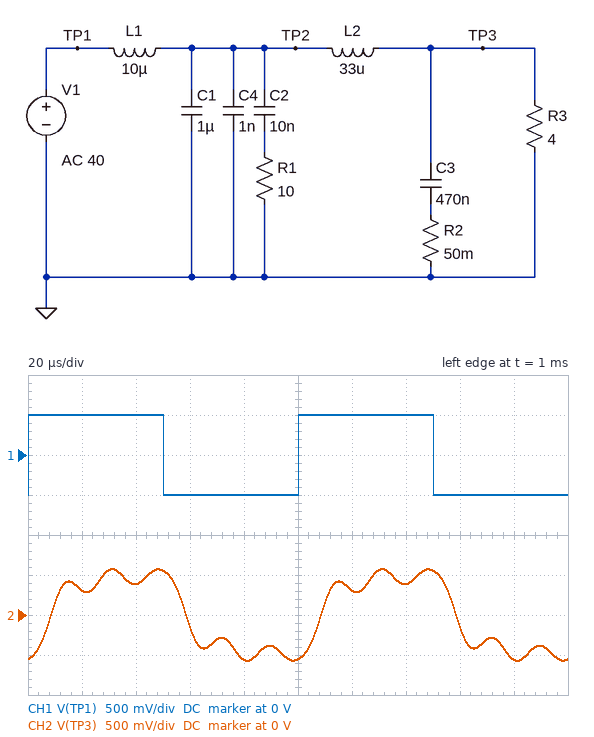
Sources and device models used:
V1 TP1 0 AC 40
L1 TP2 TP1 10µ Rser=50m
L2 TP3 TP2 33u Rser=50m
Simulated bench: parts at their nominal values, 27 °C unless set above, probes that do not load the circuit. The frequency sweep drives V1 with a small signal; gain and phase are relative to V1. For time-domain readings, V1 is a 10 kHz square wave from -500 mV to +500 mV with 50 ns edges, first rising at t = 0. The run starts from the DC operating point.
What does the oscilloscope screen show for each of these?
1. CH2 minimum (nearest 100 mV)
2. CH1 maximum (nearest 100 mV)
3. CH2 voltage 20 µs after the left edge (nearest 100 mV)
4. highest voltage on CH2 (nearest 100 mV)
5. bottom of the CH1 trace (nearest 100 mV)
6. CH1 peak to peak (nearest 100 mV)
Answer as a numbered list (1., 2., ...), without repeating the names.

1. -600 mV
2. 500 mV
3. 300 mV
4. 600 mV
5. -500 mV
6. 1.0 V
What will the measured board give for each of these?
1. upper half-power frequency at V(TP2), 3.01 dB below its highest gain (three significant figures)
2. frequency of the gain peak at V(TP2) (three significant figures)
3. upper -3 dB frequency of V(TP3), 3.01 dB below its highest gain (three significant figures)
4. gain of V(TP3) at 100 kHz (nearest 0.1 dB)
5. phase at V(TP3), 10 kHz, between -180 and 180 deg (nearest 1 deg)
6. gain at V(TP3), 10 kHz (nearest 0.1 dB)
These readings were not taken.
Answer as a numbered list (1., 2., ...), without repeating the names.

1. 60.2 kHz
2. 57.9 kHz
3. 60.0 kHz
4. -25.8 dB
5. -36 deg
6. -1.0 dB
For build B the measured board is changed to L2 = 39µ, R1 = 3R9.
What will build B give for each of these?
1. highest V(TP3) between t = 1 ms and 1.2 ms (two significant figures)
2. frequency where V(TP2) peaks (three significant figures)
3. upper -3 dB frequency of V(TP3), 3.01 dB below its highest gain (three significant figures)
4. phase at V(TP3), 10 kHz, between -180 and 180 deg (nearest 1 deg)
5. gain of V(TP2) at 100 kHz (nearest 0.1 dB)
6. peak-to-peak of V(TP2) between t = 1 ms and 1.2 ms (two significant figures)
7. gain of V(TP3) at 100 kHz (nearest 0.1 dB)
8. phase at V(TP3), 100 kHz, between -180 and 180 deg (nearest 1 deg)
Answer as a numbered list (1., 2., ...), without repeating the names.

1. 570 mV
2. 56.7 kHz
3. 58.3 kHz
4. -40 deg
5. -8.7 dB
6. 1.8 V
7. -27.6 dB
8. 46 deg
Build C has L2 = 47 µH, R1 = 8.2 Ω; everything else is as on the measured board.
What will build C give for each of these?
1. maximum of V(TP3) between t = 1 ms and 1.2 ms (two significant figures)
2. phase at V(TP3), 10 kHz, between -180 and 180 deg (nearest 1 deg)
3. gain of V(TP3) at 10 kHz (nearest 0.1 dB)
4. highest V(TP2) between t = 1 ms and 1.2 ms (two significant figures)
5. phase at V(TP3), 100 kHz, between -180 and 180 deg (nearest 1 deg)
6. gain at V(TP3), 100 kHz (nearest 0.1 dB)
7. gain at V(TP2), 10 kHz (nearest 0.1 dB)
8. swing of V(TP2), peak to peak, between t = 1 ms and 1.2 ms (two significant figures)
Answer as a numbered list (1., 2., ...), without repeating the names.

1. 570 mV
2. -45 deg
3. -1.9 dB
4. 990 mV
5. 45 deg
6. -29.5 dB
7. -0.4 dB
8. 2.0 V
